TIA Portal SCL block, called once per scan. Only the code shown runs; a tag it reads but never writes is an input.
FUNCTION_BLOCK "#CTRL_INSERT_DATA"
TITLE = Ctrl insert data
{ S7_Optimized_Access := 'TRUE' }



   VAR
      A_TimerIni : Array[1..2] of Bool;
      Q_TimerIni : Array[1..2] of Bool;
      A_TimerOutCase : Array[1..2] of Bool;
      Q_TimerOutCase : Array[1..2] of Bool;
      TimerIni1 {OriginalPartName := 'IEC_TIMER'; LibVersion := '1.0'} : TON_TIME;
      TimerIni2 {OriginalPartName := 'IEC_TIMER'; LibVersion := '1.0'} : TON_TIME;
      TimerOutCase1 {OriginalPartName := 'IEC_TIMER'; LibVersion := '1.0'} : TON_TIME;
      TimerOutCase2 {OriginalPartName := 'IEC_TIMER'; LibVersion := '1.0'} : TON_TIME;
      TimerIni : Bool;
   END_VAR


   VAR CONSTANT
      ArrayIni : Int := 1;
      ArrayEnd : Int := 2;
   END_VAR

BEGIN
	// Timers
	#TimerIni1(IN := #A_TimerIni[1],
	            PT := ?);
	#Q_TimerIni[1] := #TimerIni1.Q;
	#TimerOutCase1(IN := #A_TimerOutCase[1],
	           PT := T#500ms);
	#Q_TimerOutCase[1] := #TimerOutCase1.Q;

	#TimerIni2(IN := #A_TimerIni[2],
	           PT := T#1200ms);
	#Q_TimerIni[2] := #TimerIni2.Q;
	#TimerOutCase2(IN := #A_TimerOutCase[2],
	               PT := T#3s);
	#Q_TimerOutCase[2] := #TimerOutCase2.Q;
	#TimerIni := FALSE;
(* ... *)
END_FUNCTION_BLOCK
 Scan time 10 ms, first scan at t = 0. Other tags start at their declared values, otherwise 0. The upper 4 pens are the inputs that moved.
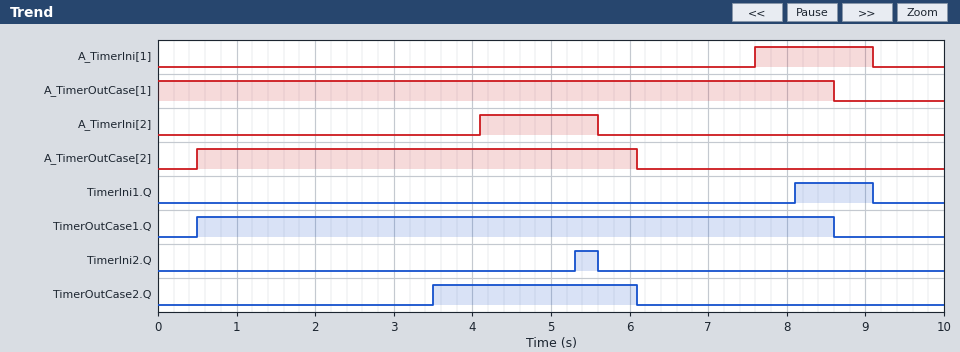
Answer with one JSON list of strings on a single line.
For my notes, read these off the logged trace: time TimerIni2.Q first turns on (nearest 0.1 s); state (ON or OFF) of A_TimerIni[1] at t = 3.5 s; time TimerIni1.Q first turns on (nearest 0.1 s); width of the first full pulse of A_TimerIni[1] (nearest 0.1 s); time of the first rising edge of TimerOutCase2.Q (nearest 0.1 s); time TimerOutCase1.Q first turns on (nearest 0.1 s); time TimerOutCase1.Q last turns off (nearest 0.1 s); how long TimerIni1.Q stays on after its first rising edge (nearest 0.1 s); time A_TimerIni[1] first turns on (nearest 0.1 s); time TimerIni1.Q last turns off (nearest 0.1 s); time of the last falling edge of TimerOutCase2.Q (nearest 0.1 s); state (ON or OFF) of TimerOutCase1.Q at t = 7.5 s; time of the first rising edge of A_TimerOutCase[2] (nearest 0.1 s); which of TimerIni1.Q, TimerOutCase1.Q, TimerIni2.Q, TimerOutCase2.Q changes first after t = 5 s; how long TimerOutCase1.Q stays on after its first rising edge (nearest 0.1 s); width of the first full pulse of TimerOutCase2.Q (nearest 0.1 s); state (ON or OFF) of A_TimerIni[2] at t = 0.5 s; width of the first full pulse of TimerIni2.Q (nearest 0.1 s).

["5.3 s", "OFF", "8.1 s", "1.5 s", "3.5 s", "0.5 s", "8.6 s", "1.0 s", "7.6 s", "9.1 s", "6.1 s", "ON", "0.5 s", "TimerIni2.Q", "8.1 s", "2.6 s", "OFF", "0.3 s"]
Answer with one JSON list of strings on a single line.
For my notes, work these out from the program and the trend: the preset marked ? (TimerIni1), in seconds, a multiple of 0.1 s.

["0.5 s"]
